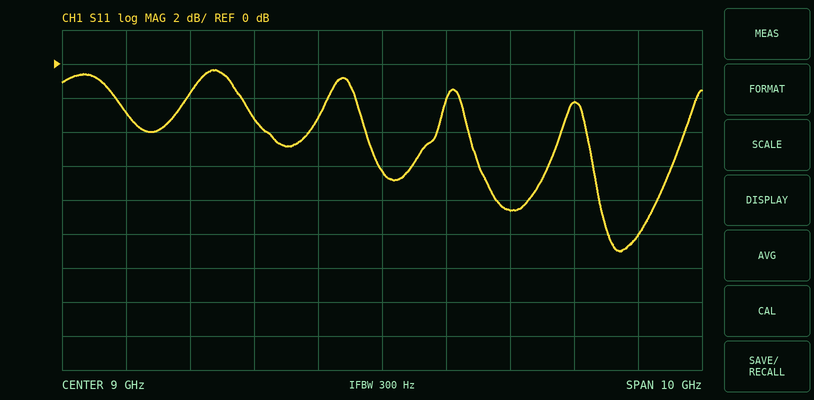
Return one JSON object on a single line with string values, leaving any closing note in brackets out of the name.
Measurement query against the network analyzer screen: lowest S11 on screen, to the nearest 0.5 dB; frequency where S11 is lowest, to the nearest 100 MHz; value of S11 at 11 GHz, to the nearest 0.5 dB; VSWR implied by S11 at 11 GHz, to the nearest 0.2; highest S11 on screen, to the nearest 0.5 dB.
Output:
{"lowest S11 on screen, to the nearest 0.5 dB": "-11.0 dB", "frequency where S11 is lowest, to the nearest 100 MHz": "12.7 GHz", "value of S11 at 11 GHz, to the nearest 0.5 dB": "-8.5 dB", "VSWR implied by S11 at 11 GHz, to the nearest 0.2": "2.2", "highest S11 on screen, to the nearest 0.5 dB": "-0.5 dB"}
